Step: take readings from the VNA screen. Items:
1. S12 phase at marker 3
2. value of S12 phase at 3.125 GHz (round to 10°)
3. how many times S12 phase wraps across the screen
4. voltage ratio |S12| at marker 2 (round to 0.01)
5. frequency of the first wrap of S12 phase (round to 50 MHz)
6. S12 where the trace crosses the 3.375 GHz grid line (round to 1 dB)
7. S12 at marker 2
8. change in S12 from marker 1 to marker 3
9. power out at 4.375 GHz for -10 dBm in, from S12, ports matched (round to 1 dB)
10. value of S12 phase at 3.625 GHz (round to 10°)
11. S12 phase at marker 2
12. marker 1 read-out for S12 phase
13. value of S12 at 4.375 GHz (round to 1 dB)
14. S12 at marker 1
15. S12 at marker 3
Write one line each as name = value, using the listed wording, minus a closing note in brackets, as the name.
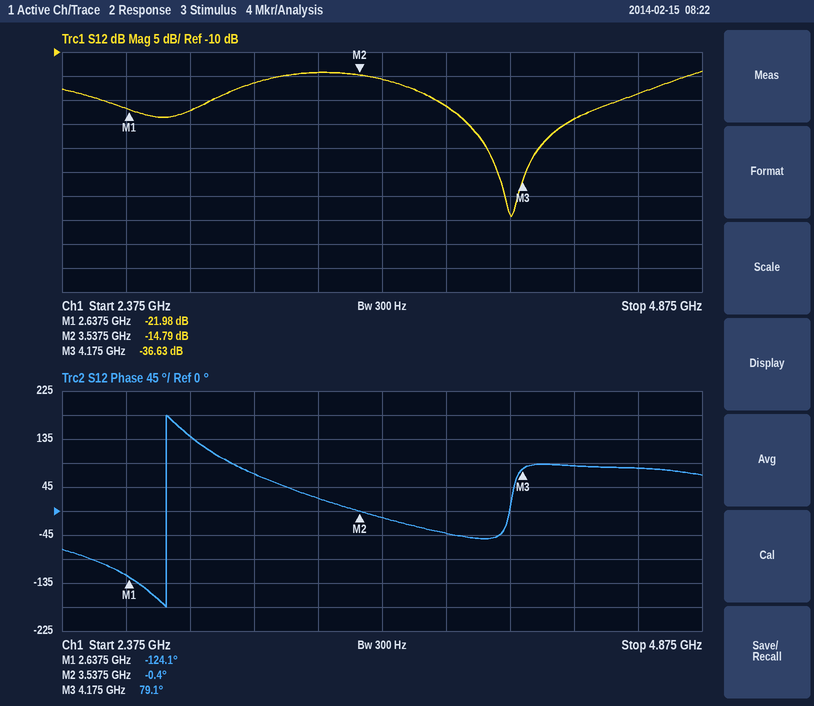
S12 phase at marker 3 = 79.1°
value of S12 phase at 3.125 GHz = 70°
how many times S12 phase wraps across the screen = 1
voltage ratio |S12| at marker 2 = 0.18
frequency of the first wrap of S12 phase = 2.80 GHz
S12 where the trace crosses the 3.375 GHz grid line = -14 dB
S12 at marker 2 = -14.79 dB
change in S12 from marker 1 to marker 3 = -14.65 dB
power out at 4.375 GHz for -10 dBm in, from S12, ports matched = -34 dBm
value of S12 phase at 3.625 GHz = -10°
S12 phase at marker 2 = -0.4°
marker 1 read-out for S12 phase = -124.1°
value of S12 at 4.375 GHz = -24 dB
S12 at marker 1 = -21.98 dB
S12 at marker 3 = -36.63 dB
